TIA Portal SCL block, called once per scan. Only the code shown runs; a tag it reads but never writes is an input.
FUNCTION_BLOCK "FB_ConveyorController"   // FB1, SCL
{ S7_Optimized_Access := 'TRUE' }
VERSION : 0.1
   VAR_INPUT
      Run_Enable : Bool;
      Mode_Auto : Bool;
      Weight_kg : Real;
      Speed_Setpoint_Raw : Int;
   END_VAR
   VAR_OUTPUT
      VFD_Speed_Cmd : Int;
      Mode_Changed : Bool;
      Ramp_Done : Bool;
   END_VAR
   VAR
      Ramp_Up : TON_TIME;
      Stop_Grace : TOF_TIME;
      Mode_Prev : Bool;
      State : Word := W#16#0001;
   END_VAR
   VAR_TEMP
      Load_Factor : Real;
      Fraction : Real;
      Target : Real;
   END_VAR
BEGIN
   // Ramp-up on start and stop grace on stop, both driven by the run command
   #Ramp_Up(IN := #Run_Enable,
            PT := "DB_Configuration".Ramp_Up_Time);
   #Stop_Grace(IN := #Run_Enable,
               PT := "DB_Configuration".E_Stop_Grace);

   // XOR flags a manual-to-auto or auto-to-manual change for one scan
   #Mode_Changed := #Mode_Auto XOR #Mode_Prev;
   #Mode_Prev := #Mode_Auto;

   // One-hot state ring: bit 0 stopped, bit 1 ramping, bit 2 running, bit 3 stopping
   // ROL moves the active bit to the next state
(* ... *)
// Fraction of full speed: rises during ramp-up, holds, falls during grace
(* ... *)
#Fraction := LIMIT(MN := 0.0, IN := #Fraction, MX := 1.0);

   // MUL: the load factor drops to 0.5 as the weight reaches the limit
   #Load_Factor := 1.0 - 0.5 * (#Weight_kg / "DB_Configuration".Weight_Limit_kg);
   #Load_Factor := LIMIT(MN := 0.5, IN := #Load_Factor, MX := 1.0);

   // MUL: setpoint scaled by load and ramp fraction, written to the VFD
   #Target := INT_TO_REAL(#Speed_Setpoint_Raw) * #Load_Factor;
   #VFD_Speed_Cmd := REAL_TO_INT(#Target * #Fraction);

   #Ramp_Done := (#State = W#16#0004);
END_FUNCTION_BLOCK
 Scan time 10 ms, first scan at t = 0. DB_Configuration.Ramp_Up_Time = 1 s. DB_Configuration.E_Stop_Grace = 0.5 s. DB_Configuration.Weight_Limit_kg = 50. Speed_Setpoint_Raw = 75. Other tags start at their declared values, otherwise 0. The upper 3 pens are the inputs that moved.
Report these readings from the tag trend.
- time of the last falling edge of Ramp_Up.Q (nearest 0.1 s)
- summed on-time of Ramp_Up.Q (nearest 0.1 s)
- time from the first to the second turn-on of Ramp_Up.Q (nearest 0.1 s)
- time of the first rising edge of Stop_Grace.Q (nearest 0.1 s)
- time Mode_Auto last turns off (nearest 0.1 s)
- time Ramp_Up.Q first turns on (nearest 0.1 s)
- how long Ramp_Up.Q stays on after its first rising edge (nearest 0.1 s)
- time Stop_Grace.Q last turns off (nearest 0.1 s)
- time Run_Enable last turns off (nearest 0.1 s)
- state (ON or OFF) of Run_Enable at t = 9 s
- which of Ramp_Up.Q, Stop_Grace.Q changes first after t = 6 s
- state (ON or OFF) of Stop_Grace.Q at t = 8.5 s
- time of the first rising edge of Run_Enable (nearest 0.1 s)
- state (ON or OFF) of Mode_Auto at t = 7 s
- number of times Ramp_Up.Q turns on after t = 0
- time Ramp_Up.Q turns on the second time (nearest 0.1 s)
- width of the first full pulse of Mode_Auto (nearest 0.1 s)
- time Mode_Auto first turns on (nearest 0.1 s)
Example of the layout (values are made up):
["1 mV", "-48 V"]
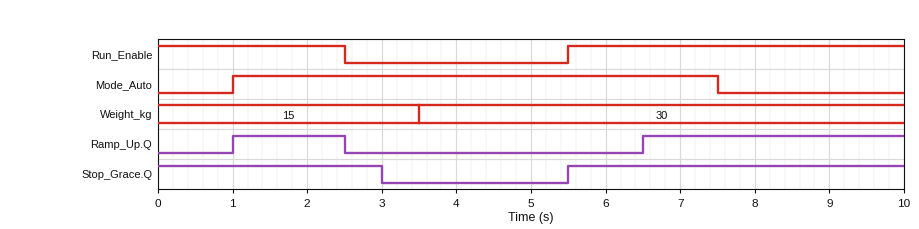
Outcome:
["2.5 s", "5.0 s", "5.5 s", "5.5 s", "7.5 s", "1.0 s", "1.5 s", "3.0 s", "2.5 s", "ON", "Ramp_Up.Q", "ON", "5.5 s", "ON", "2", "6.5 s", "6.5 s", "1.0 s"]
